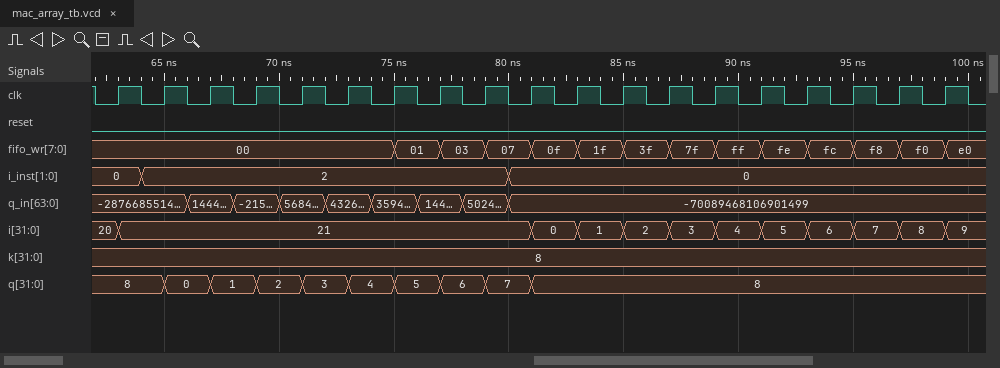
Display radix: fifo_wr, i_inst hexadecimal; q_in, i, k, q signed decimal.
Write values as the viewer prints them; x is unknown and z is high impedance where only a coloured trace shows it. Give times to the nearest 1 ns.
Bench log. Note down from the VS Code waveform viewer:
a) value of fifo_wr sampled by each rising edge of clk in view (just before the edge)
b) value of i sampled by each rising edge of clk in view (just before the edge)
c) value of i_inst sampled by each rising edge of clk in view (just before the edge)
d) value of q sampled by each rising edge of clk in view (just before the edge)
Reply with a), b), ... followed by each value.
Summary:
a) 00, 00, 00, 00, 00, 00, 00, 01, 03, 07, 0f, 1f, 3f, 7f, ff, fe, fc, f8, f0
b) 20, 21, 21, 21, 21, 21, 21, 21, 21, 21, 0, 1, 2, 3, 4, 5, 6, 7, 8
c) 0, 2, 2, 2, 2, 2, 2, 2, 2, 0, 0, 0, 0, 0, 0, 0, 0, 0, 0
d) 8, 8, 0, 1, 2, 3, 4, 5, 6, 7, 8, 8, 8, 8, 8, 8, 8, 8, 8
